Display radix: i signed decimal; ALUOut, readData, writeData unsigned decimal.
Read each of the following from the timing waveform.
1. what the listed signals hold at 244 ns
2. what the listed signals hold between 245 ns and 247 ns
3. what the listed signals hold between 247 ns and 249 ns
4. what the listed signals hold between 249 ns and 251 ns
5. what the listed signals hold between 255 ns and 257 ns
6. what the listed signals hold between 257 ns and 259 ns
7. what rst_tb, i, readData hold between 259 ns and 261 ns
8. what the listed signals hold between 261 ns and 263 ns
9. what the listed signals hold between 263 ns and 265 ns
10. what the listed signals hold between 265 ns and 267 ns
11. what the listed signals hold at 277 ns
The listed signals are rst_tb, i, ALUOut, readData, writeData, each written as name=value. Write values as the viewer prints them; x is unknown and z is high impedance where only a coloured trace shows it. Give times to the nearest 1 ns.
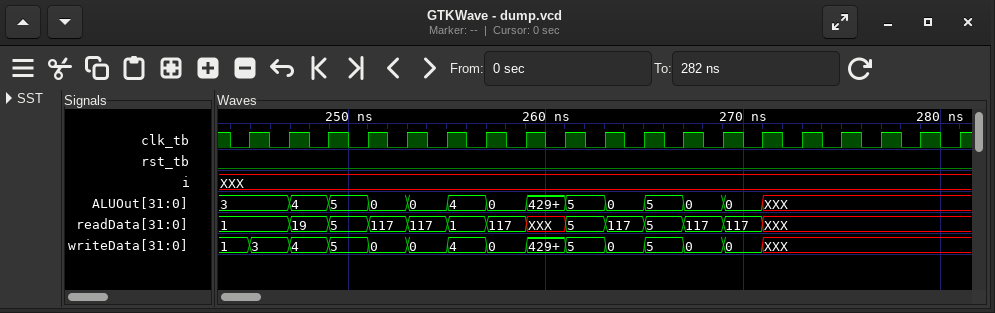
rst_tb=0, i=XXX, ALUOut=3, readData=1, writeData=1
rst_tb=0, i=XXX, ALUOut=3, readData=1, writeData=3
rst_tb=0, i=XXX, ALUOut=4, readData=19, writeData=4
rst_tb=0, i=XXX, ALUOut=5, readData=5, writeData=5
rst_tb=0, i=XXX, ALUOut=4, readData=1, writeData=4
rst_tb=0, i=XXX, ALUOut=0, readData=117, writeData=0
rst_tb=0, i=XXX, readData=XXX
rst_tb=0, i=XXX, ALUOut=5, readData=5, writeData=5
rst_tb=0, i=XXX, ALUOut=0, readData=117, writeData=0
rst_tb=0, i=XXX, ALUOut=5, readData=5, writeData=5
rst_tb=0, i=XXX, ALUOut=XXX, readData=XXX, writeData=XXX
